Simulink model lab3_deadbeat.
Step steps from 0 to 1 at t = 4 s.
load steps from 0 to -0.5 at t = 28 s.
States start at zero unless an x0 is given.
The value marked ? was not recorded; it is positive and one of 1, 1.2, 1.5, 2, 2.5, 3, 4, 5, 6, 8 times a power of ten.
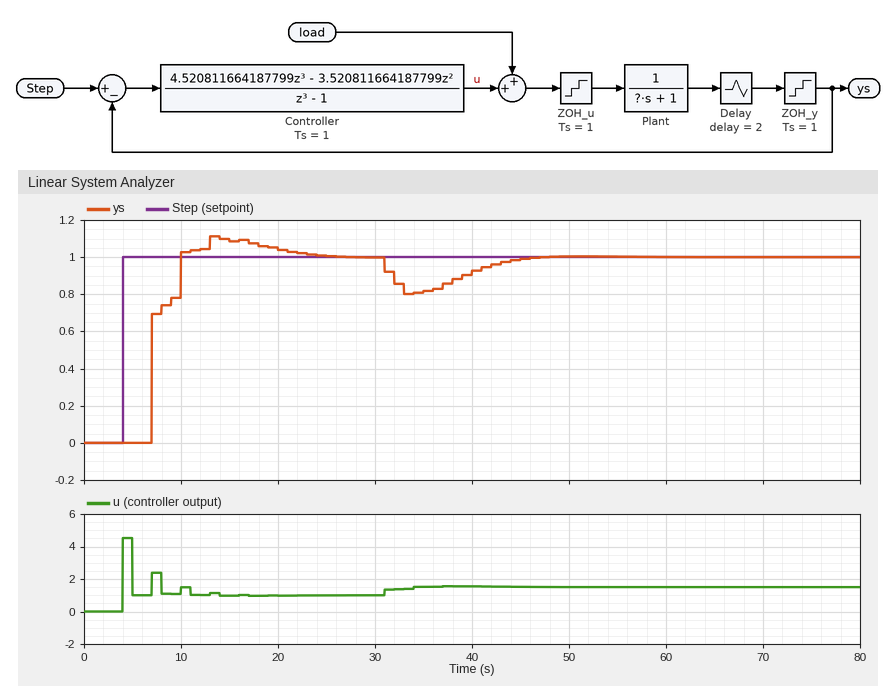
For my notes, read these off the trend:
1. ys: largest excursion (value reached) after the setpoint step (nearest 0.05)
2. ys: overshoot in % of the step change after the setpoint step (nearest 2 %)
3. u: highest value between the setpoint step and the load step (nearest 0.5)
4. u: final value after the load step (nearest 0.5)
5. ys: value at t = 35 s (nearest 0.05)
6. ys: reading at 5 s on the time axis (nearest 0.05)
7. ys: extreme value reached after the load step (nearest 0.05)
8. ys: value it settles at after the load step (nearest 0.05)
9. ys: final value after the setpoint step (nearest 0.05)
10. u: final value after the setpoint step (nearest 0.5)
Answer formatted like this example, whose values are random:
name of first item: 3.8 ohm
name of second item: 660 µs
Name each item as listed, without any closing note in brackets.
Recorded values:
ys: largest excursion (value reached) after the setpoint step: 1.10
ys: overshoot in % of the step change after the setpoint step: 12 %
u: highest value between the setpoint step and the load step: 4.5
u: final value after the load step: 1.5
ys: value at t = 35 s: 0.80
ys: reading at 5 s on the time axis: 0.00
ys: extreme value reached after the load step: 0.80
ys: value it settles at after the load step: 1.00
ys: final value after the setpoint step: 1.00
u: final value after the setpoint step: 1.0
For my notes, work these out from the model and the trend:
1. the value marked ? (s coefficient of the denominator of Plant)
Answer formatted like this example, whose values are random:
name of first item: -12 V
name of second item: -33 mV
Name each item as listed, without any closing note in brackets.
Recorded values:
the value marked ?: 6
